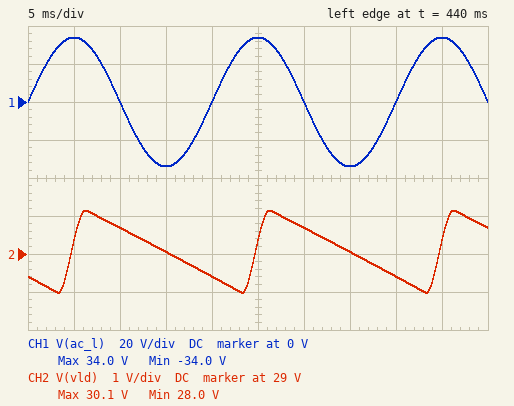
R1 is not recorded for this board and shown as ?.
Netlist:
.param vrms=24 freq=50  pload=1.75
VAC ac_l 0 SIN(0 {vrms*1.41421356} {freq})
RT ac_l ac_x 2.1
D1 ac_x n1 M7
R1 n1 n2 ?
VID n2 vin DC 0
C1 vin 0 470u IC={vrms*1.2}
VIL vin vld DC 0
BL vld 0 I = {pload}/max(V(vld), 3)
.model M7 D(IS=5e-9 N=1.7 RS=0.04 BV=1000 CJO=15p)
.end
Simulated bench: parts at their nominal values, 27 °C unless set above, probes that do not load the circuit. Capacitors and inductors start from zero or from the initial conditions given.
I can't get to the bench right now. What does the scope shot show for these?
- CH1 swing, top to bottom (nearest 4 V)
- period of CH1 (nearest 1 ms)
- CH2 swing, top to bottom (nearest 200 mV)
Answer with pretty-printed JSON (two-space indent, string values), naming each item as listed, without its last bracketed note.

{
  "CH1 swing, top to bottom": "68 V",
  "period of CH1": "20 ms",
  "CH2 swing, top to bottom": "2.2 V"
}
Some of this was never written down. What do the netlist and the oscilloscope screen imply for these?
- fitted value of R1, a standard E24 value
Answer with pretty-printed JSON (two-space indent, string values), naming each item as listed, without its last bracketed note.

{
  "fitted value of R1, a standard E24 value": "4.7 Ω"
}
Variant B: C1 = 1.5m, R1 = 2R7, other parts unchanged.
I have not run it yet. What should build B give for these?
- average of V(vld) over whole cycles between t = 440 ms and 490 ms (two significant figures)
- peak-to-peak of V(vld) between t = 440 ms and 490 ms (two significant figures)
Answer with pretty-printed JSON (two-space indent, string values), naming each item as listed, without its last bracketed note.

{
  "average of V(vld) over whole cycles between t = 440 ms and 490 ms": "30 V",
  "peak-to-peak of V(vld) between t = 440 ms and 490 ms": "670 mV"
}
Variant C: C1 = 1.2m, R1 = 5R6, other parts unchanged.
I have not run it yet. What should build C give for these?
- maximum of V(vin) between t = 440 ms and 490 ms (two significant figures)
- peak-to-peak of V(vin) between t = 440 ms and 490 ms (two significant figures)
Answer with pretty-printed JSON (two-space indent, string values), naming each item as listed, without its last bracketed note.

{
  "maximum of V(vin) between t = 440 ms and 490 ms": "29 V",
  "peak-to-peak of V(vin) between t = 440 ms and 490 ms": "850 mV"
}
